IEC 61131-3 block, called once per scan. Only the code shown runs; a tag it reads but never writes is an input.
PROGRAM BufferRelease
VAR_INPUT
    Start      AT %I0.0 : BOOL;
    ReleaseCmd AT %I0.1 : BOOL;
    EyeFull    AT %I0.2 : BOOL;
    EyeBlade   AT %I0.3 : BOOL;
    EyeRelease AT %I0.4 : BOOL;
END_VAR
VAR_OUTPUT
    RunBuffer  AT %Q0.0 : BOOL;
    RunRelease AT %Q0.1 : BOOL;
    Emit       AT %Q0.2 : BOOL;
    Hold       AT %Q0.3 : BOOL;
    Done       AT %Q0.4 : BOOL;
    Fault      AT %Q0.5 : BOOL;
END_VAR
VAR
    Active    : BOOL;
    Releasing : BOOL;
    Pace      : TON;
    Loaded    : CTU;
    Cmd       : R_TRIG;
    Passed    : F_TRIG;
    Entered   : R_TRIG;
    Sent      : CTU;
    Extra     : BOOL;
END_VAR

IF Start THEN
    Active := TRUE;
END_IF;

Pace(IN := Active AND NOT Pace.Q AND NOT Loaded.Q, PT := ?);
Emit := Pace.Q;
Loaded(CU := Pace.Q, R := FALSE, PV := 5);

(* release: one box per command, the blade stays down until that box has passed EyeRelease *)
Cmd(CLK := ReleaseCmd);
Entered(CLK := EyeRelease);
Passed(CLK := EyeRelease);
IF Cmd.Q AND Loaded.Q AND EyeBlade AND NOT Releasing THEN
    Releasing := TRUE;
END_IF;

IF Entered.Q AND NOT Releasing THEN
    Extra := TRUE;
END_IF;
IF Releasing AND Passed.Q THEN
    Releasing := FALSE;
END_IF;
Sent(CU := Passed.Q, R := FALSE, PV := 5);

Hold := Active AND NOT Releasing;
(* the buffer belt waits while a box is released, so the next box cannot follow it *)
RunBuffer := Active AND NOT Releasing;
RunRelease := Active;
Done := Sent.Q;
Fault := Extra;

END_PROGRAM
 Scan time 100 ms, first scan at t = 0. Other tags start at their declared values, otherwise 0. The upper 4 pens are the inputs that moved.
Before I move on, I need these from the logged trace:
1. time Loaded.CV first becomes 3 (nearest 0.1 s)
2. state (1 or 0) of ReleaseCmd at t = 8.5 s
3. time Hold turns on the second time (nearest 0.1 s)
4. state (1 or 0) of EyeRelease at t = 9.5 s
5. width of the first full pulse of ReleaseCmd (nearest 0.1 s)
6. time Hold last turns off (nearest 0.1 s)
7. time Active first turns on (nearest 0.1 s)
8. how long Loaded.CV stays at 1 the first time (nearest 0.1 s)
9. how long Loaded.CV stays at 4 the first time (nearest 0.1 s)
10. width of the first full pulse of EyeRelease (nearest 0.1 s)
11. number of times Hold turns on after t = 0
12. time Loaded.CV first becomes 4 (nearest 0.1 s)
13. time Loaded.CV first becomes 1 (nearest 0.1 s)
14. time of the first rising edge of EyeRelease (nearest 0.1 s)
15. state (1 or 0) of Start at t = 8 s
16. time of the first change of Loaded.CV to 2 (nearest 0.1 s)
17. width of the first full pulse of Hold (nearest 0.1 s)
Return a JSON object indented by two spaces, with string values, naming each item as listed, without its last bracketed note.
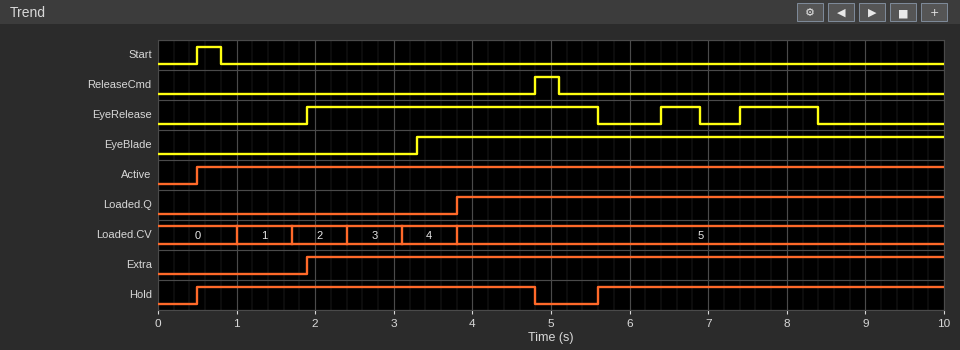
{
  "time Loaded.CV first becomes 3": "2.4 s",
  "state (1 or 0) of ReleaseCmd at t = 8.5 s": "0",
  "time Hold turns on the second time": "5.6 s",
  "state (1 or 0) of EyeRelease at t = 9.5 s": "0",
  "width of the first full pulse of ReleaseCmd": "0.3 s",
  "time Hold last turns off": "4.8 s",
  "time Active first turns on": "0.5 s",
  "how long Loaded.CV stays at 1 the first time": "0.7 s",
  "how long Loaded.CV stays at 4 the first time": "0.7 s",
  "width of the first full pulse of EyeRelease": "3.7 s",
  "number of times Hold turns on after t = 0": "2",
  "time Loaded.CV first becomes 4": "3.1 s",
  "time Loaded.CV first becomes 1": "1.0 s",
  "time of the first rising edge of EyeRelease": "1.9 s",
  "state (1 or 0) of Start at t = 8 s": "0",
  "time of the first change of Loaded.CV to 2": "1.7 s",
  "width of the first full pulse of Hold": "4.3 s"
}
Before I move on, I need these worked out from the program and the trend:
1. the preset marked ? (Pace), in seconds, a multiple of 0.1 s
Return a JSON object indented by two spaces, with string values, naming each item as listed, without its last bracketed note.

{
  "the preset marked ? (Pace), in seconds, a multiple of 0.1 s": "0.5 s"
}
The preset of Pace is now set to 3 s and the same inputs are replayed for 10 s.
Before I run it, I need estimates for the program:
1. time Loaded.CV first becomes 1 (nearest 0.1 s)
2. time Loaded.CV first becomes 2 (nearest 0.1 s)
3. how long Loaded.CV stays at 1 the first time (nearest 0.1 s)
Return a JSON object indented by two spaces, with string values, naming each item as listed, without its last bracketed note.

{
  "time Loaded.CV first becomes 1": "3.5 s",
  "time Loaded.CV first becomes 2": "6.7 s",
  "how long Loaded.CV stays at 1 the first time": "3.2 s"
}
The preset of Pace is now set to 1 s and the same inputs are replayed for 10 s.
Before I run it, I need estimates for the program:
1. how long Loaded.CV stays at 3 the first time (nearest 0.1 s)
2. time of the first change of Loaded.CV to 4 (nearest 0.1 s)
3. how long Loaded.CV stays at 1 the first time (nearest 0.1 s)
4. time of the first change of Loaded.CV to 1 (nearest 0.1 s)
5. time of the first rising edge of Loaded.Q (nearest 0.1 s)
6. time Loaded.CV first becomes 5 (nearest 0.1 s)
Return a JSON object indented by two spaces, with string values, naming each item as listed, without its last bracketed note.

{
  "how long Loaded.CV stays at 3 the first time": "1.2 s",
  "time of the first change of Loaded.CV to 4": "5.1 s",
  "how long Loaded.CV stays at 1 the first time": "1.2 s",
  "time of the first change of Loaded.CV to 1": "1.5 s",
  "time of the first rising edge of Loaded.Q": "6.3 s",
  "time Loaded.CV first becomes 5": "6.3 s"
}
